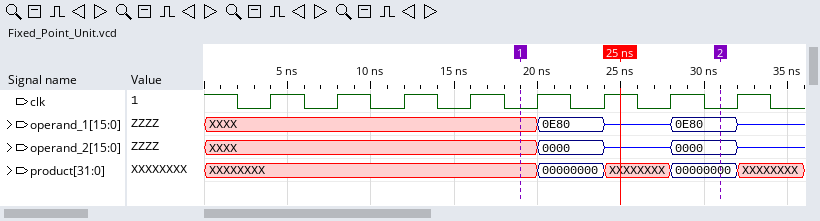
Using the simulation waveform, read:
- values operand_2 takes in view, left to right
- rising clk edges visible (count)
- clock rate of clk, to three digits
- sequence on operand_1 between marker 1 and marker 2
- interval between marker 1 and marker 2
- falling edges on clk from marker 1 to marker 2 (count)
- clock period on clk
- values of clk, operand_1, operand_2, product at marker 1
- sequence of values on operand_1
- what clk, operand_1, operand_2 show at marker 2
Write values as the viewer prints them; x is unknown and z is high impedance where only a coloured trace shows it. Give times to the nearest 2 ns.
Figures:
XXXX, 0000, z, 0000, z
8
250 MHz
XXXX, 0E80, z, 0E80
12 ns
3
4 ns
clk=0, operand_1=XXXX, operand_2=XXXX, product=XXXXXXXX
XXXX, 0E80, z, 0E80, z
clk=0, operand_1=0E80, operand_2=0000
